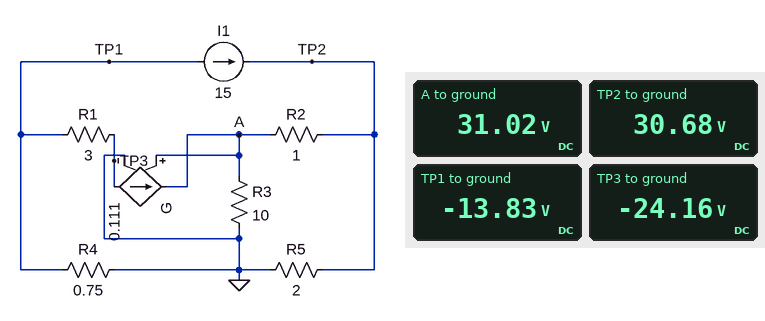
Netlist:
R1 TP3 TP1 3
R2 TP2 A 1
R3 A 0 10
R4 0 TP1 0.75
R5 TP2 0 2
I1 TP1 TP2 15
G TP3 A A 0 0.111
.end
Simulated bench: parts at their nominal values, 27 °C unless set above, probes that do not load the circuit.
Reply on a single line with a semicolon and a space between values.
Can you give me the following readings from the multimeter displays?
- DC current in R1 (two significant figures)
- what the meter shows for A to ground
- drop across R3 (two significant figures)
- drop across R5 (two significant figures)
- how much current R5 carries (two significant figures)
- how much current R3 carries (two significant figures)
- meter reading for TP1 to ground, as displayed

3.4 A; 31.02 V; 31 V; 31 V; 15 A; 3.1 A; -13.83 V
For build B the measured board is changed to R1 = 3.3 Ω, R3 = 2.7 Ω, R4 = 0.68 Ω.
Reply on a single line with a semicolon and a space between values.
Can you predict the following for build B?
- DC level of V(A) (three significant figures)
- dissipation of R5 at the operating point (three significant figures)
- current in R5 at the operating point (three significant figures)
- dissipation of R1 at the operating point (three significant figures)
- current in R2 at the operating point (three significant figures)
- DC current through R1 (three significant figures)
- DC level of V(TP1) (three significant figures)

16.9 V; 226 W; 10.6 A; 11.6 W; 4.38 A; 1.87 A; -11.5 V
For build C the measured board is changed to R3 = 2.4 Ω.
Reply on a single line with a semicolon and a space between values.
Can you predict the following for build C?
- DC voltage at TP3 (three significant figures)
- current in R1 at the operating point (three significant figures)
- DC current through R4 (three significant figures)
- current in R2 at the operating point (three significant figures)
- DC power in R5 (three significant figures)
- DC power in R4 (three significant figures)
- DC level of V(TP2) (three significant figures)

-17.8 V; 1.74 A; 16.7 A; 4.78 A; 209 W; 210 W; 20.4 V
